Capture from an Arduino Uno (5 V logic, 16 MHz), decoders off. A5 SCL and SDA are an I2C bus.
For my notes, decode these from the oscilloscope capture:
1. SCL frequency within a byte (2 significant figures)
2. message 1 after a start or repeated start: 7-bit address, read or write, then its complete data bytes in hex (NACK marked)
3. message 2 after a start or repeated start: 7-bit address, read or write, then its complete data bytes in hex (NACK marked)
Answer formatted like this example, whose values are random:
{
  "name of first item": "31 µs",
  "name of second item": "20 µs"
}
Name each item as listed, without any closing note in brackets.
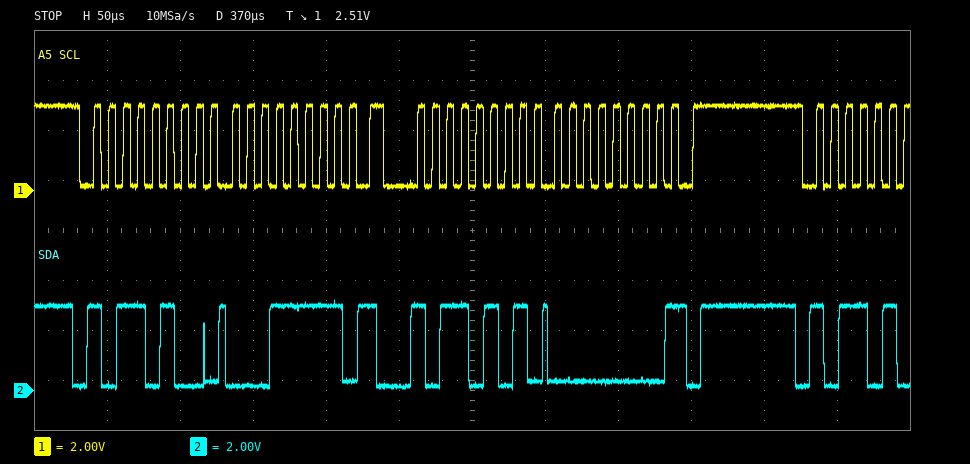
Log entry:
{
  "SCL frequency within a byte": "100 kHz",
  "message 1 after a start or repeated start: 7-bit address, read or write, then its complete data bytes in hex": "0x5A write: 1F",
  "message 2 after a start or repeated start: 7-bit address, read or write, then its complete data bytes in hex": "0x5A read: 00 NACK"
}
